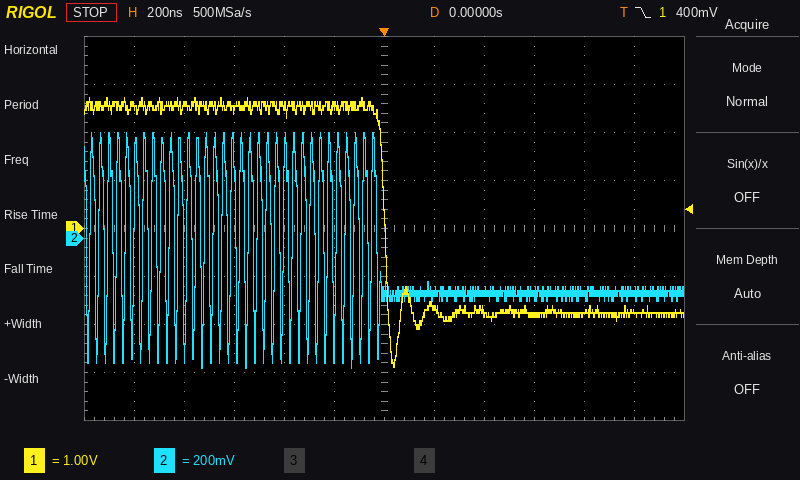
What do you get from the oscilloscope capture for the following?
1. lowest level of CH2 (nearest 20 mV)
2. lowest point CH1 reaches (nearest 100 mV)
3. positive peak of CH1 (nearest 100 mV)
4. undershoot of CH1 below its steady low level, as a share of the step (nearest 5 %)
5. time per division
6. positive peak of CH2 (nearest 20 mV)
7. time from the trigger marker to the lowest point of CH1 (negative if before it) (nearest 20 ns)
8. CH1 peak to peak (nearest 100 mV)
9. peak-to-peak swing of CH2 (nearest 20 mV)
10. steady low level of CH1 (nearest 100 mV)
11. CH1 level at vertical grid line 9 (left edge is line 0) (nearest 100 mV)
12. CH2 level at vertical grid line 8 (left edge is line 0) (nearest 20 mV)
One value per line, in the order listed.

-540 mV
-2.9 V
2.7 V
25 %
200 ns
440 mV
+40 ns
5.6 V
980 mV
-1.8 V
-1.8 V
-220 mV
